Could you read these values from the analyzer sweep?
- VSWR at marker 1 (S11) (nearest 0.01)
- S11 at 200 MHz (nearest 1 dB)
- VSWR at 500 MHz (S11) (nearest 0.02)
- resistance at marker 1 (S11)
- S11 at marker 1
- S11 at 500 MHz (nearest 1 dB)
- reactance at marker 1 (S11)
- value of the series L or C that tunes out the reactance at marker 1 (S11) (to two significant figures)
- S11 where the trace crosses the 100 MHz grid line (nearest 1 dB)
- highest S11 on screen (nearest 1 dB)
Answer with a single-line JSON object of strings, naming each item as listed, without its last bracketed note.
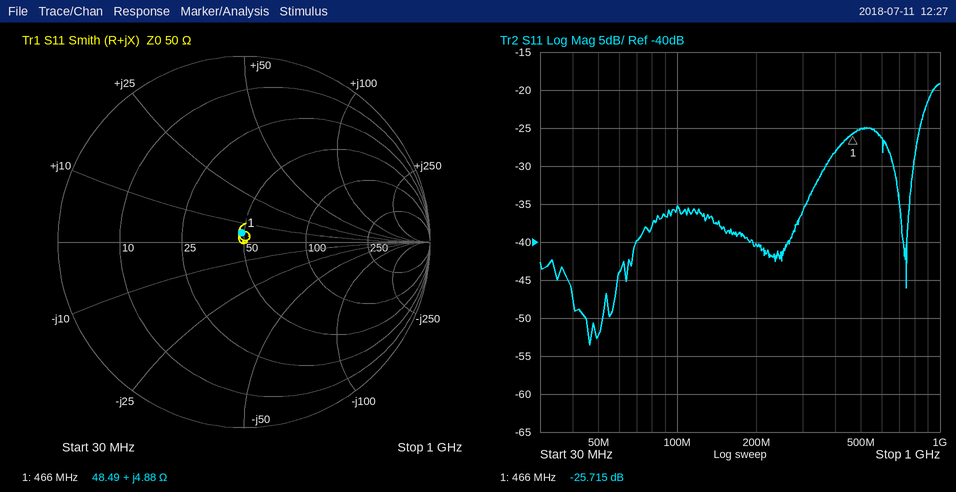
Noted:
{"VSWR at marker 1 (S11)": "1.11", "S11 at 200 MHz": "-40 dB", "VSWR at 500 MHz (S11)": "1.12", "resistance at marker 1": "48.49 Ω", "S11 at marker 1": "-25.715 dB", "S11 at 500 MHz": "-25 dB", "reactance at marker 1": "+4.88 Ω", "value of the series L or C that tunes out the reactance at marker 1 (S11)": "70 pF", "S11 where the trace crosses the 100 MHz grid line": "-35 dB", "highest S11 on screen": "-19 dB"}
